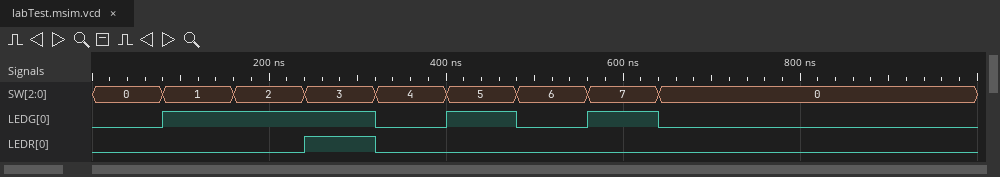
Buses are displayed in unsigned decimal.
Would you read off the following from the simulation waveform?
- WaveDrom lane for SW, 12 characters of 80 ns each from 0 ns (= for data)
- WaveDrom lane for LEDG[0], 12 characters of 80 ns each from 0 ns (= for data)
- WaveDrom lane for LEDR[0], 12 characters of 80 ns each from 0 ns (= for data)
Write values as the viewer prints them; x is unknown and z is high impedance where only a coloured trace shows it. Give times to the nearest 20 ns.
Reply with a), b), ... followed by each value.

a) {name: 'SW', wave: '=========...', data: '0 1 2 3 4 5 6 7 0'}
b) {name: 'LEDG[0]', wave: '01..01010...'}
c) {name: 'LEDR[0]', wave: '0..10.......'}
